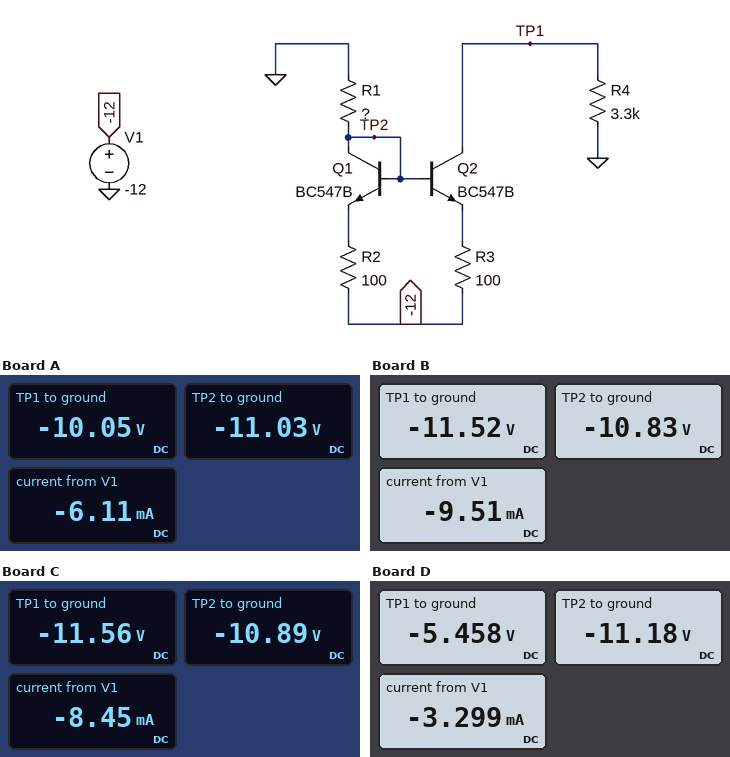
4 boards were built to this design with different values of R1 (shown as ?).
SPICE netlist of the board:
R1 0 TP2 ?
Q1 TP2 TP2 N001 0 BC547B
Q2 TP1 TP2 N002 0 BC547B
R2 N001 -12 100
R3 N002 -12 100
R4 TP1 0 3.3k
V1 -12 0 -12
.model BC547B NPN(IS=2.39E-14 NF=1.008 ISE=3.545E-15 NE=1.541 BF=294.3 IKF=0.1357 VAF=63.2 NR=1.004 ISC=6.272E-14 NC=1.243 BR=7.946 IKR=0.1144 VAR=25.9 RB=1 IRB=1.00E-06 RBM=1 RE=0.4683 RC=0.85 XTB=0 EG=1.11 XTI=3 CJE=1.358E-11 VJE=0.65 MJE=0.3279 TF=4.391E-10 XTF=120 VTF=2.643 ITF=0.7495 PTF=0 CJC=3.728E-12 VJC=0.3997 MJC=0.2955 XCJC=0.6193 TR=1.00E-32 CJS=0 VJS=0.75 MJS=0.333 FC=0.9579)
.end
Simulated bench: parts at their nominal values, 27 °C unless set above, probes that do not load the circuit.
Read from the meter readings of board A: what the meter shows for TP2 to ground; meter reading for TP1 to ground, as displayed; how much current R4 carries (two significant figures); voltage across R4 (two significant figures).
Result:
-11.03 V
-10.05 V
3.0 mA
10 V
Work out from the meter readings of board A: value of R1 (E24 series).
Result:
3.6 kΩ
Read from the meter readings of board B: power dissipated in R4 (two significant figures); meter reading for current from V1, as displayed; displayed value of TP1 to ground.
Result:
40 mW
-9.51 mA
-11.52 V
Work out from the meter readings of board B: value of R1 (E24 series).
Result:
1.8 kΩ
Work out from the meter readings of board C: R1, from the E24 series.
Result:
2.2 kΩ
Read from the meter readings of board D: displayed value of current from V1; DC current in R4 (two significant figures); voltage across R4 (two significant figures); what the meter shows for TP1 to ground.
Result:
-3.299 mA
1.7 mA
5.5 V
-5.458 V
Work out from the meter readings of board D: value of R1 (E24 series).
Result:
6.8 kΩ
